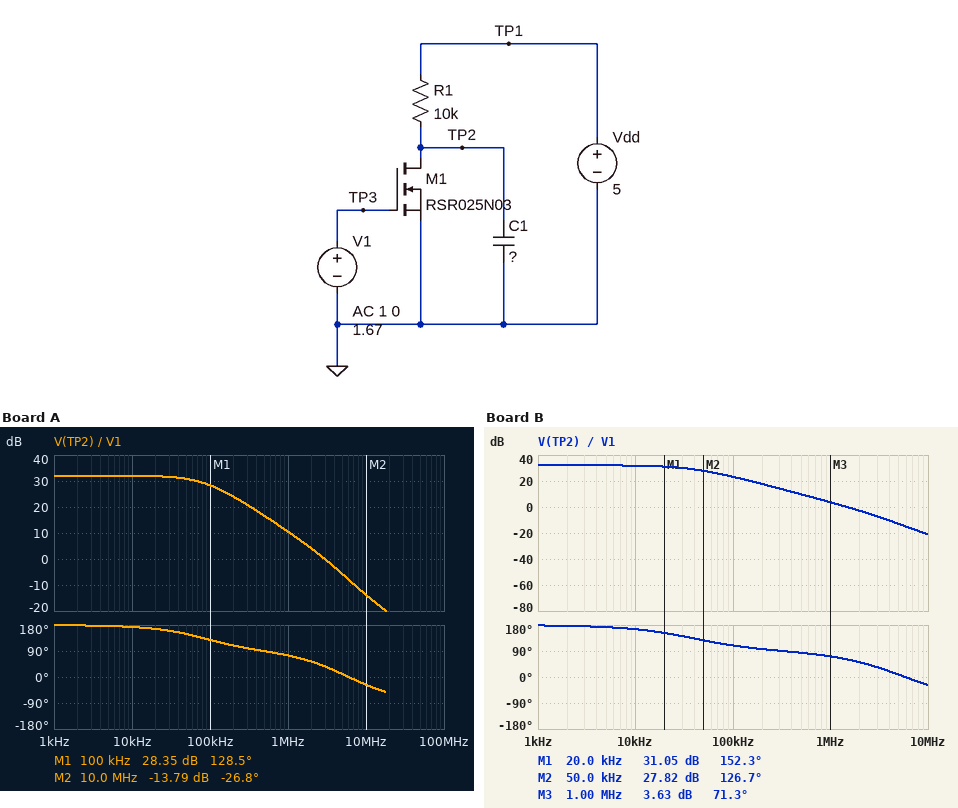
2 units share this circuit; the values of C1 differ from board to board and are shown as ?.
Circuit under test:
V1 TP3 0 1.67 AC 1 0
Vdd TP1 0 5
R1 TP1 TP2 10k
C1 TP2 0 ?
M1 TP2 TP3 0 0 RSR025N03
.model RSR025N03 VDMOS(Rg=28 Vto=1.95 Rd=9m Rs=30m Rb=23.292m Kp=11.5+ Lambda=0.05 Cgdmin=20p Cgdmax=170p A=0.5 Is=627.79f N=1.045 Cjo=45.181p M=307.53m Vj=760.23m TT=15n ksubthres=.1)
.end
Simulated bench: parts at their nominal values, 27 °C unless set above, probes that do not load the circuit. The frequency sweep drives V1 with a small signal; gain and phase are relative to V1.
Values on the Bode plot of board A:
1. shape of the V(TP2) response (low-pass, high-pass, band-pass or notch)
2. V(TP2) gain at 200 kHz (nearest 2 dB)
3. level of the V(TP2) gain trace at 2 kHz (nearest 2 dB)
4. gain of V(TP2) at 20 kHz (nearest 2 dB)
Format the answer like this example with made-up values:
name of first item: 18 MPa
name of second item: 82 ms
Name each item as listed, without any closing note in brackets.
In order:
shape of the V(TP2) response: low-pass
V(TP2) gain at 200 kHz: 24 dB
level of the V(TP2) gain trace at 2 kHz: 32 dB
gain of V(TP2) at 20 kHz: 32 dB
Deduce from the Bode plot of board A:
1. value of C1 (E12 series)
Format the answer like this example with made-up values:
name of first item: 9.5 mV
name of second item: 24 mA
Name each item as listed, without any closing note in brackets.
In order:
value of C1: 82 pF
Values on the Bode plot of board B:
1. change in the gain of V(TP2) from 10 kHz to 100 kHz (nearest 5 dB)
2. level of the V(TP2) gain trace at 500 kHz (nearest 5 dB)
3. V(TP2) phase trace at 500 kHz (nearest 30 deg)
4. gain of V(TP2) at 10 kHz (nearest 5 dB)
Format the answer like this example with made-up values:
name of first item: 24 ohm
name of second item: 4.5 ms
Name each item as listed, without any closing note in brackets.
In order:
change in the gain of V(TP2) from 10 kHz to 100 kHz: -10 dB
level of the V(TP2) gain trace at 500 kHz: 10 dB
V(TP2) phase trace at 500 kHz: 90 deg
gain of V(TP2) at 10 kHz: 30 dB
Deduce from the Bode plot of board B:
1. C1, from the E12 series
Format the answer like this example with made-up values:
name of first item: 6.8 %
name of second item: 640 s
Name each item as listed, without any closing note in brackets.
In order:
C1, from the E12 series: 330 pF
